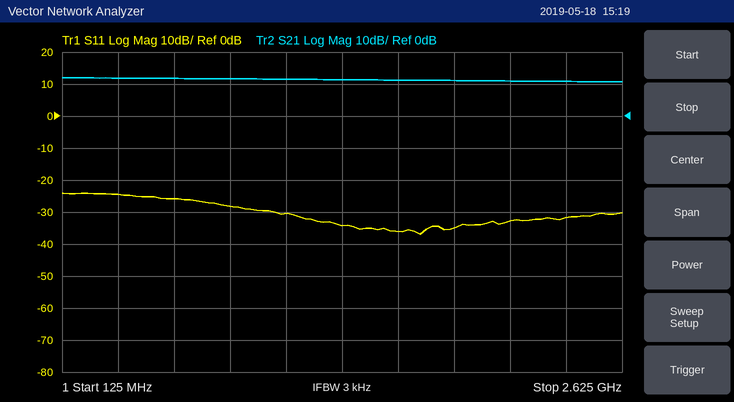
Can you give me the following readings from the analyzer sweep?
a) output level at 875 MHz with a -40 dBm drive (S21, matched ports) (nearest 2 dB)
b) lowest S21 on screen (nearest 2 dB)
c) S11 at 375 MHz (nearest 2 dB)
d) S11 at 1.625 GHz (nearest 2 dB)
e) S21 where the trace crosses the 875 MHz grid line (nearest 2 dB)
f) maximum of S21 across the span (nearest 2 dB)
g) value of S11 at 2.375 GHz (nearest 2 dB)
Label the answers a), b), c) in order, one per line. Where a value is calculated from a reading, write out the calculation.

a) -40 dBm + (12 dB) = -28 dBm
b) 10 dB
c) -24 dB
d) -36 dB
e) 12 dB
f) 12 dB
g) -32 dB
